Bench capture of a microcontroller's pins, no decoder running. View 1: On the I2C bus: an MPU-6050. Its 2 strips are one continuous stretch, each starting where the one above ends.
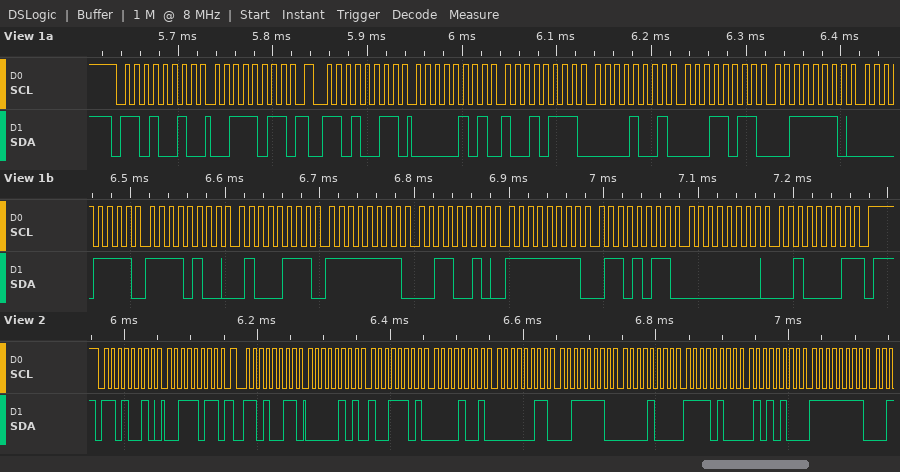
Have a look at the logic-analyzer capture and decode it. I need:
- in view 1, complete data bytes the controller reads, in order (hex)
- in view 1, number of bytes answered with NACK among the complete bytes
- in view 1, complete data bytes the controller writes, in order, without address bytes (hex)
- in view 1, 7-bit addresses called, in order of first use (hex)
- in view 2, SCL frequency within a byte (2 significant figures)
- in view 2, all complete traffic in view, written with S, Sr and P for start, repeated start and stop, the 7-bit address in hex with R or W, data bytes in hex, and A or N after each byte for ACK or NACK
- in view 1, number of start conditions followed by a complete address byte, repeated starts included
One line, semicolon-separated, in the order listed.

05 97 09 1B 3E 0F F4 47 FF 32 FF 6B 00 21; 1; 3B; 0x69; 100 kHz; S 69W A 3B A Sr 69R A 05 A 9D A 09 A 03 A 3E A 08 A F4 A 54 A FF A; 2
